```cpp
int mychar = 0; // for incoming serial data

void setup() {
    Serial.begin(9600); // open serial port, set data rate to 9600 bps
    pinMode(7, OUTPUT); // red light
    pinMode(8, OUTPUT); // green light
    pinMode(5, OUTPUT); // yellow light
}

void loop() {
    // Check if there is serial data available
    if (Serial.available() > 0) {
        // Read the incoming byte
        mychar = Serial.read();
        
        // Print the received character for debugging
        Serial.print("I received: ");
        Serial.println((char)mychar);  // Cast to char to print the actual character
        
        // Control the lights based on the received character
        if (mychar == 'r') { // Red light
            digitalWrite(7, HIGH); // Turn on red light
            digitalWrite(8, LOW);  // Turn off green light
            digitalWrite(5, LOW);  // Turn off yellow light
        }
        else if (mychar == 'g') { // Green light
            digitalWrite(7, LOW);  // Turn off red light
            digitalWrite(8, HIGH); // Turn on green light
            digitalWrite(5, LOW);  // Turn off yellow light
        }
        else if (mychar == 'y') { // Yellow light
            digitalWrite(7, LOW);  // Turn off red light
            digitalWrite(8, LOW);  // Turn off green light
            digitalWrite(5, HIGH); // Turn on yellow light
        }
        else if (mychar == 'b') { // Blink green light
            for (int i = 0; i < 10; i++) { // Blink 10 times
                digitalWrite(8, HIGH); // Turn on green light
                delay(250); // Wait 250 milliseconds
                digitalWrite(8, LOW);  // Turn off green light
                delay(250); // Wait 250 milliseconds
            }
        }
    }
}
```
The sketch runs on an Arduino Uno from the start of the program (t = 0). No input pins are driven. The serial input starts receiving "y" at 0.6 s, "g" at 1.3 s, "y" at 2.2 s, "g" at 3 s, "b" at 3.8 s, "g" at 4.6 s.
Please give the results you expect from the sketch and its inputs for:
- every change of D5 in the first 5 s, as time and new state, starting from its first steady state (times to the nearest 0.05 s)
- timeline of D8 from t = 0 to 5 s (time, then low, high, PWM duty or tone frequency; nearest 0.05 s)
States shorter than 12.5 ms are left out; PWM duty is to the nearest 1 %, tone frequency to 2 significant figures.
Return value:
0 s low; 0.6 s high; 1.3 s low; 2.2 s high; 3 s low
0 s low; 1.3 s high; 2.2 s low; 3 s high; 4.05 s low; 4.3 s high; 4.55 s low; 4.8 s high
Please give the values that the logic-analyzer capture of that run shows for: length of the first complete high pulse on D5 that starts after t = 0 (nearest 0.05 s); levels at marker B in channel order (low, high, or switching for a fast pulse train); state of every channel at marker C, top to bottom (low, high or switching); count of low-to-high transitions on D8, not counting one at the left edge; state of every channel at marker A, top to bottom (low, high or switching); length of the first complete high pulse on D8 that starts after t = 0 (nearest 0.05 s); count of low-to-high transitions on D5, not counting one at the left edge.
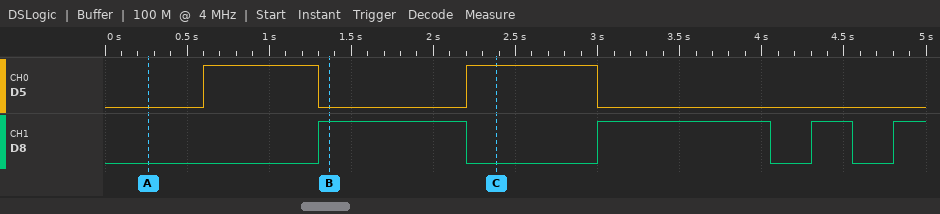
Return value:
0.70 s
D5 low, D8 high
D5 high, D8 low
4
D5 low, D8 low
0.90 s
2
